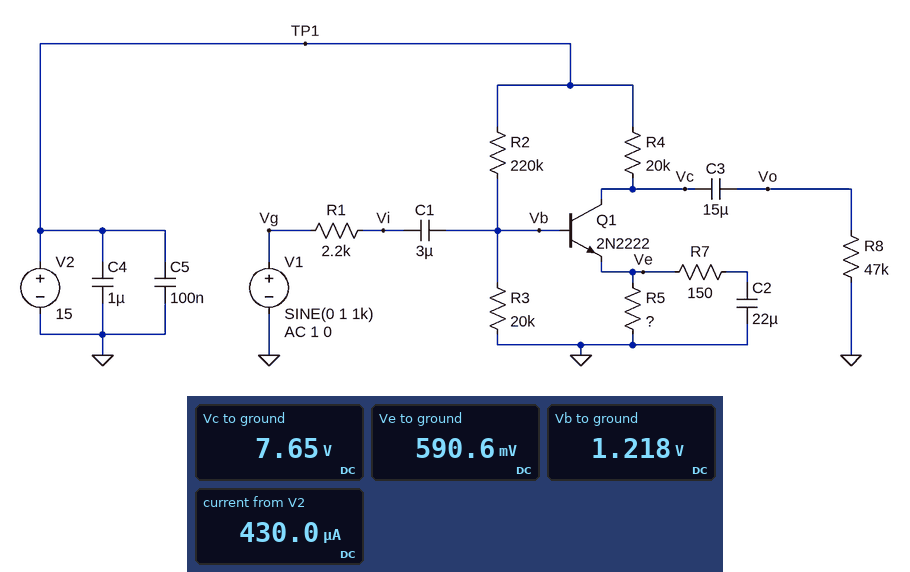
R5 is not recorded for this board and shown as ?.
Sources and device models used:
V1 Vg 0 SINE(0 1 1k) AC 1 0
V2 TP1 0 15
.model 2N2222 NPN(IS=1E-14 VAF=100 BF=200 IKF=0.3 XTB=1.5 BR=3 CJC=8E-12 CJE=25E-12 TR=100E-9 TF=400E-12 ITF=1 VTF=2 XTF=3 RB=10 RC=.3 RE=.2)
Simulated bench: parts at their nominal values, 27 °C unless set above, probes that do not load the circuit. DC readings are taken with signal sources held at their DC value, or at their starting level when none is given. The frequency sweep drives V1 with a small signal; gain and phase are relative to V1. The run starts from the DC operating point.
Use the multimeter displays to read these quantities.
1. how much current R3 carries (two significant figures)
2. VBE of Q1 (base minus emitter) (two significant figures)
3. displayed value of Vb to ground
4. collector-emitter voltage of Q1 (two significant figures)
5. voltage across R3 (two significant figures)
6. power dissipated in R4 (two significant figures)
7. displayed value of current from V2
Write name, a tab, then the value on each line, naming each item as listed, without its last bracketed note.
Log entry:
how much current R3 carries	61 µA
VBE of Q1 (base minus emitter)	630 mV
displayed value of Vb to ground	1.218 V
collector-emitter voltage of Q1	7.1 V
voltage across R3	1.2 V
power dissipated in R4	2.7 mW
displayed value of current from V2	430.0 µA
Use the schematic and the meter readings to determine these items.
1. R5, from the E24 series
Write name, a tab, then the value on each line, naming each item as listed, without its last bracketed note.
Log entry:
R5, from the E24 series	1.6 kΩ
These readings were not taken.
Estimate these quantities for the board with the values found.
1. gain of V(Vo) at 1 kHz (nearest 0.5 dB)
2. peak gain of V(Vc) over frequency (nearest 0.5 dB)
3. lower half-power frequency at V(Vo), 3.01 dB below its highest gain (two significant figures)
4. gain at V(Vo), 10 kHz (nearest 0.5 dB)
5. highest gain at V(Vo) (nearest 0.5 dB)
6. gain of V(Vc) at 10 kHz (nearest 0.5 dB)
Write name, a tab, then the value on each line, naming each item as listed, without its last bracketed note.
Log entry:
gain of V(Vo) at 1 kHz	35.0 dB
peak gain of V(Vc) over frequency	35.0 dB
lower half-power frequency at V(Vo), 3.01 dB below its highest gain	32 Hz
gain at V(Vo), 10 kHz	35.0 dB
highest gain at V(Vo)	35.0 dB
gain of V(Vc) at 10 kHz	35.0 dB
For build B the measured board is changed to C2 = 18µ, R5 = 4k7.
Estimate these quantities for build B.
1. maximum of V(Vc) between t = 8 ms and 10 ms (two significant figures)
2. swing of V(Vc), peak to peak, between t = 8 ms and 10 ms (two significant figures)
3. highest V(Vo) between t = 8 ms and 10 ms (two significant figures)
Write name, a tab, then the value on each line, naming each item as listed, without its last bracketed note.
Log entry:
maximum of V(Vc) between t = 8 ms and 10 ms	14 V
swing of V(Vc), peak to peak, between t = 8 ms and 10 ms	13 V
highest V(Vo) between t = 8 ms and 10 ms	1.9 V
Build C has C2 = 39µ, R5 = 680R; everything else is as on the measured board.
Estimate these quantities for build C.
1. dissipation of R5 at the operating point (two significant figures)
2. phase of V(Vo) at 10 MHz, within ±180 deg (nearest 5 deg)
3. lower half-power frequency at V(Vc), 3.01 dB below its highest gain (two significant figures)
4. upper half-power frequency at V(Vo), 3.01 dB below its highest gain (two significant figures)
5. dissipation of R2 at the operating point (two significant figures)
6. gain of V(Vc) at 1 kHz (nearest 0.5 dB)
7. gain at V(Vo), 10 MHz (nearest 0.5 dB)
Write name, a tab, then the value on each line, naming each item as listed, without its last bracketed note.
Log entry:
dissipation of R5 at the operating point	360 µW
phase of V(Vo) at 10 MHz, within ±180 deg	65 deg
lower half-power frequency at V(Vc), 3.01 dB below its highest gain	23 Hz
upper half-power frequency at V(Vo), 3.01 dB below its highest gain	410 kHz
dissipation of R2 at the operating point	870 µW
gain of V(Vc) at 1 kHz	12.0 dB
gain at V(Vo), 10 MHz	-15.0 dB
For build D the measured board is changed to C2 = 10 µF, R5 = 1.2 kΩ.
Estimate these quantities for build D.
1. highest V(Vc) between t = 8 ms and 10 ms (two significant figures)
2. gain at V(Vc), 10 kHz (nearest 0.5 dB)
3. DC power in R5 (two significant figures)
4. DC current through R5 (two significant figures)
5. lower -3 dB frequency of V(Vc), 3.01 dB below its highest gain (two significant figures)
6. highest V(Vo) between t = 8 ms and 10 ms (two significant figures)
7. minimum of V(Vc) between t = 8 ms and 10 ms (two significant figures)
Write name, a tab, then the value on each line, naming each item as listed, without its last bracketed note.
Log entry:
highest V(Vc) between t = 8 ms and 10 ms	12 V
gain at V(Vc), 10 kHz	36.0 dB
DC power in R5	270 µW
DC current through R5	480 µA
lower -3 dB frequency of V(Vc), 3.01 dB below its highest gain	73 Hz
highest V(Vo) between t = 8 ms and 10 ms	6.7 V
minimum of V(Vc) between t = 8 ms and 10 ms	660 mV
